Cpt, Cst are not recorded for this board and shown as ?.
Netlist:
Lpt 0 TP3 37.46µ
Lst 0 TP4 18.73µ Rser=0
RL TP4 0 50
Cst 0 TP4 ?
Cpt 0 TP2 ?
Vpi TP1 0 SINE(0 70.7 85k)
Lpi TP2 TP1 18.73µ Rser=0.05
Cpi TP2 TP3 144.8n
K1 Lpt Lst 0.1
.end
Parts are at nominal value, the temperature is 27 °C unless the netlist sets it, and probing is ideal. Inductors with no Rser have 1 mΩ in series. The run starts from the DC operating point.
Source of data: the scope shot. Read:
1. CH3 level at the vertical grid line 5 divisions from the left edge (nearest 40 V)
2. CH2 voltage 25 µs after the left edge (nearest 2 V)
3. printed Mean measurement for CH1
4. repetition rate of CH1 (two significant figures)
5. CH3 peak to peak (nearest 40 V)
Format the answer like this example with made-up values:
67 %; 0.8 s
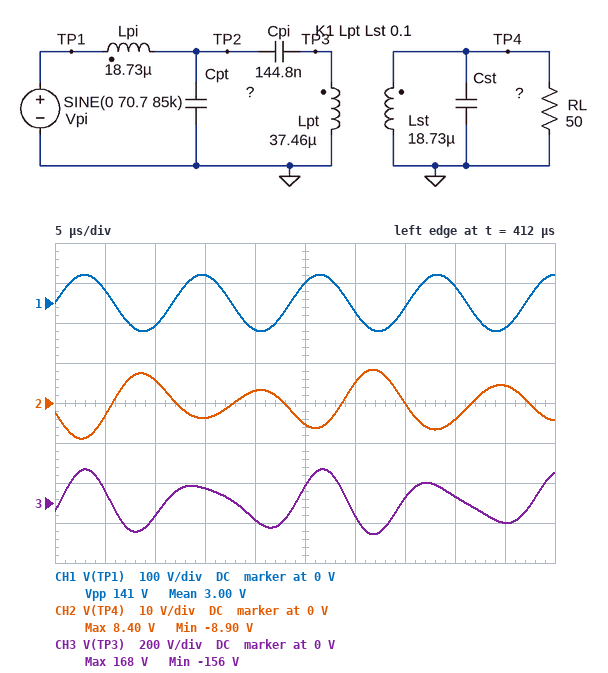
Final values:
80 V; -6 V; 3.00 V; 85 kHz; 320 V
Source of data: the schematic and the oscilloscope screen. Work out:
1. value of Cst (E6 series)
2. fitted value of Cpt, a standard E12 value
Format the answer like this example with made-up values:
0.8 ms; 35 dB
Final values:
470 nF; 150 nF
